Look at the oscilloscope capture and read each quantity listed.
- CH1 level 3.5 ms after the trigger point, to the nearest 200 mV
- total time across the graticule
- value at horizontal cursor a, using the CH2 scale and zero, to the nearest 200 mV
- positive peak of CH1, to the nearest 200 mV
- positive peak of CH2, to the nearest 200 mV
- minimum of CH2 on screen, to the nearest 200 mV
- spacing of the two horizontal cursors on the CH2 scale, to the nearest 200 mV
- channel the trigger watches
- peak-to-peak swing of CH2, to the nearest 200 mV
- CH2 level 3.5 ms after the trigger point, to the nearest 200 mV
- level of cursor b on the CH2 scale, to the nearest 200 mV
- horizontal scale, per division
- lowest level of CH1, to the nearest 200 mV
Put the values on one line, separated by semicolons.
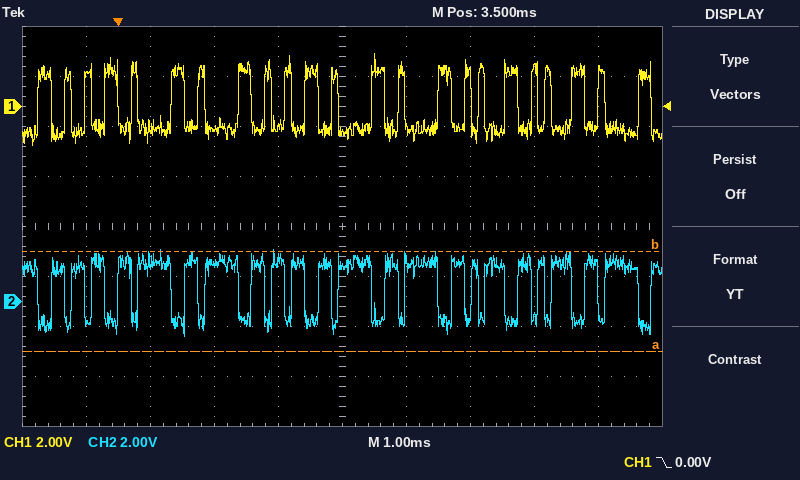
-1.0 V; 10 ms; -2.0 V; 2.2 V; 2.0 V; -1.4 V; 4.0 V; CH1; 3.4 V; 1.4 V; 2.0 V; 1 ms; -1.6 V
